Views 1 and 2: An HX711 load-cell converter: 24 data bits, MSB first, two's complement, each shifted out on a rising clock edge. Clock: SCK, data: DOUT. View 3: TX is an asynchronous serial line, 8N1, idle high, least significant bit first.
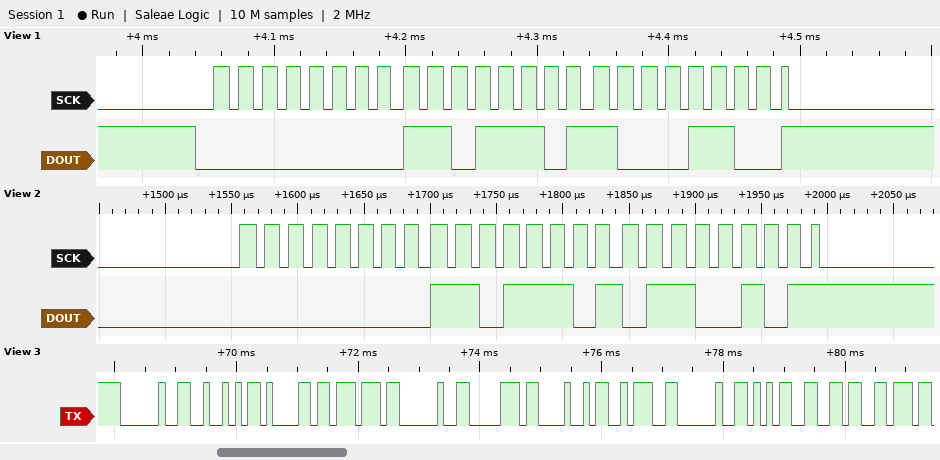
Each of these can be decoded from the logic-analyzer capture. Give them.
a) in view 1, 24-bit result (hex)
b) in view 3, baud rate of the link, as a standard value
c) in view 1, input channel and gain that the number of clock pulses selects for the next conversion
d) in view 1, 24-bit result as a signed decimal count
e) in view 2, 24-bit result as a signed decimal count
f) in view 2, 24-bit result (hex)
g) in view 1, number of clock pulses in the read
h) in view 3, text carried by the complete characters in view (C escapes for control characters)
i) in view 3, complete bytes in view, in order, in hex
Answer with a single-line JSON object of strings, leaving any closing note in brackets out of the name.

{"in view 1, 24-bit result": "0x00DD8C", "in view 3, baud rate of the link, as a standard value": "9600 baud", "in view 1, input channel and gain that the number of clock pulses selects for the next conversion": "channel A, gain 128", "in view 1, 24-bit result as a signed decimal count": "56716", "in view 2, 24-bit result as a signed decimal count": "56677", "in view 2, 24-bit result": "0x00DD65", "in view 1, number of clock pulses in the read": "25", "in view 3, text carried by the complete characters in view": "\" Raw pH: 56\"", "in view 3, complete bytes in view, in order, in hex": "20 52 61 77 20 70 48 3A 20 35 36"}
